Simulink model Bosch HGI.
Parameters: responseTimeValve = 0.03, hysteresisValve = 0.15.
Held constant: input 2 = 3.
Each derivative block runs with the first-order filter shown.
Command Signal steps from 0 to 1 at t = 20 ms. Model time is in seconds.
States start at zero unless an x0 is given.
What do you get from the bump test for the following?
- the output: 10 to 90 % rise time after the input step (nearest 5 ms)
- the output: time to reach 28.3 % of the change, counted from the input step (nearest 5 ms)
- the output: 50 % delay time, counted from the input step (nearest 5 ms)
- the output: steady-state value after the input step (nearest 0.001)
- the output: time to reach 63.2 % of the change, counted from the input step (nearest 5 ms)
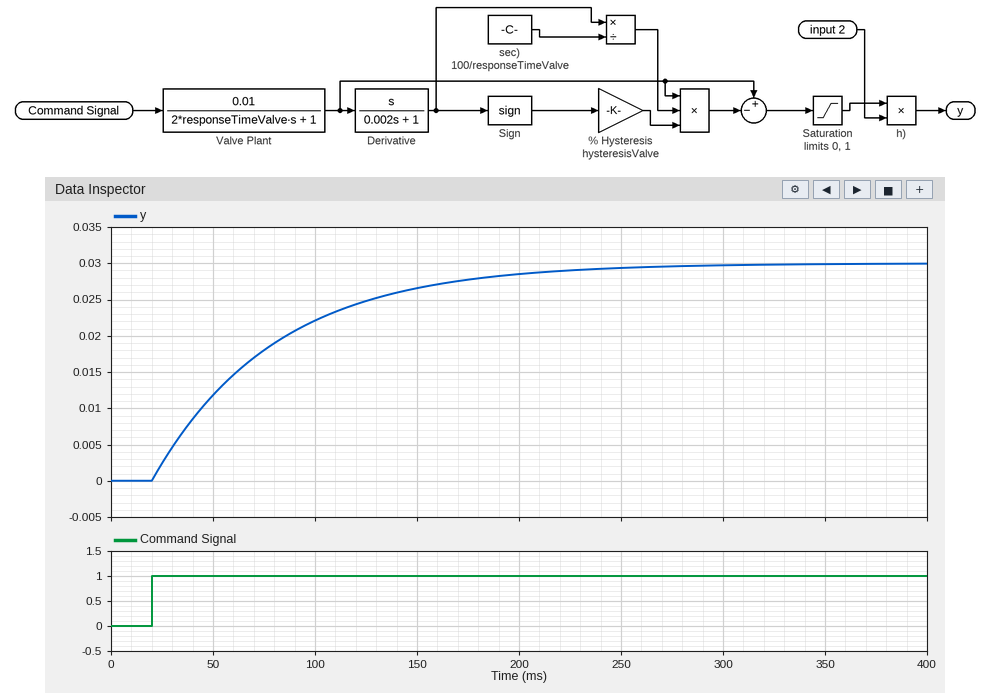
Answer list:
130 ms
20 ms
40 ms
0.030
60 ms
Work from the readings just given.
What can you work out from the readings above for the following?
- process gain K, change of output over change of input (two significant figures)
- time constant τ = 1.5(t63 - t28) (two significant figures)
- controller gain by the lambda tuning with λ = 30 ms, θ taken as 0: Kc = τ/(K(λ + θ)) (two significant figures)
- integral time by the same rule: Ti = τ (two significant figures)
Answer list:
0.030
60 ms
67
60 ms
